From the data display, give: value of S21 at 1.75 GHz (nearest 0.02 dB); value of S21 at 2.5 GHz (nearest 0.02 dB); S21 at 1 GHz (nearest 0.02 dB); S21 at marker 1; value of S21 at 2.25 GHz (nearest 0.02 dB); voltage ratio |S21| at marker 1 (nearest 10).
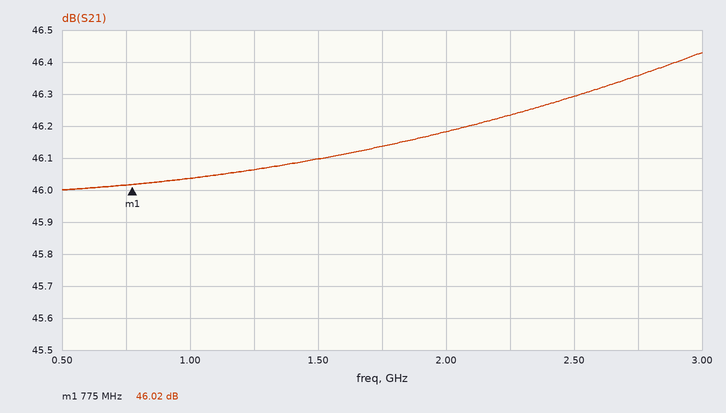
46.14 dB
46.30 dB
46.04 dB
46.02 dB
46.24 dB
200
